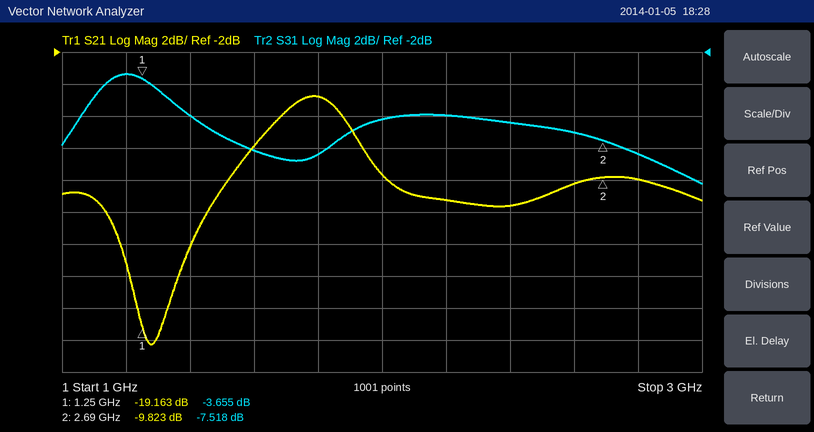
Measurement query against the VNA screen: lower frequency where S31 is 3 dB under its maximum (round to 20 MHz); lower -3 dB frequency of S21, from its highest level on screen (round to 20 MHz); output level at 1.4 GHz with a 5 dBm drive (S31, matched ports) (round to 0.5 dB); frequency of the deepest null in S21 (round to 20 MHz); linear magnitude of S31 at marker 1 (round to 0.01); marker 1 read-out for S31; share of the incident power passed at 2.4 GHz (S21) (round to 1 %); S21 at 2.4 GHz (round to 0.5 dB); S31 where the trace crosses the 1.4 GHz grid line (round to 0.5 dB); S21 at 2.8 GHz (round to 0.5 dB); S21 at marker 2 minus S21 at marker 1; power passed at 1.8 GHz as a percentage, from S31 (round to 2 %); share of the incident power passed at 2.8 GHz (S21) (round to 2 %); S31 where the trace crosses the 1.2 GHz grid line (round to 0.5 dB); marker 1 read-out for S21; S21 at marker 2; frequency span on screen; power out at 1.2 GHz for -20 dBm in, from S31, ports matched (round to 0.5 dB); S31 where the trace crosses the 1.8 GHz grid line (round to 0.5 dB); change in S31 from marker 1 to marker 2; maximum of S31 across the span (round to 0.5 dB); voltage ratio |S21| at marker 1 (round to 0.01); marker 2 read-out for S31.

1.04 GHz
1.60 GHz
-1.0 dBm
1.28 GHz
0.66
-3.655 dB
7 %
-11.5 dB
-6.0 dB
-10.0 dB
9.340 dB
14 %
10 %
-3.5 dB
-19.163 dB
-9.823 dB
2 GHz
-23.5 dBm
-8.5 dB
-3.863 dB
-3.5 dB
0.11
-7.518 dB
